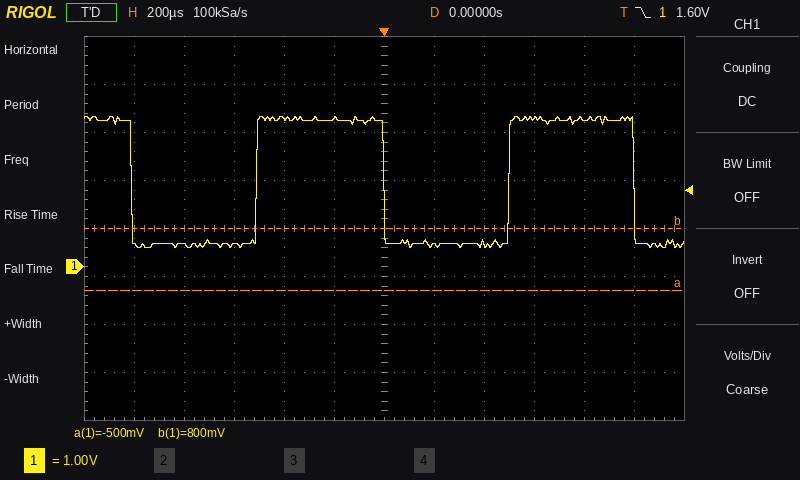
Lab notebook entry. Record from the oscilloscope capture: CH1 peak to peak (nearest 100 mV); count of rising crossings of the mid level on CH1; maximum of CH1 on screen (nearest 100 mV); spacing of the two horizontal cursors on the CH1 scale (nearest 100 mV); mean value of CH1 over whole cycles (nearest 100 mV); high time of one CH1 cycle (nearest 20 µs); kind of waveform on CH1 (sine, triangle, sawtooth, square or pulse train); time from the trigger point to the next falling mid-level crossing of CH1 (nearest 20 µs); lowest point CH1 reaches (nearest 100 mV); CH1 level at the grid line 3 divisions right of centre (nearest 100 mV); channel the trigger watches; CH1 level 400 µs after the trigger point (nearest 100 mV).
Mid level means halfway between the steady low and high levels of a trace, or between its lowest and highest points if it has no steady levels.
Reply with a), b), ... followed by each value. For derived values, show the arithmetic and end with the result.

a) 3.1 V − (400 mV) = 2.7 V
b) 2
c) 3.1 V
d) 1.3 V
e) 400 mV + 0.5 × (3.1 V − (400 mV)) ≈ 1.8 V
f) 500 µs
g) square
h) 1.00 ms
i) 400 mV
j) 3.1 V
k) CH1
l) 500 mV
